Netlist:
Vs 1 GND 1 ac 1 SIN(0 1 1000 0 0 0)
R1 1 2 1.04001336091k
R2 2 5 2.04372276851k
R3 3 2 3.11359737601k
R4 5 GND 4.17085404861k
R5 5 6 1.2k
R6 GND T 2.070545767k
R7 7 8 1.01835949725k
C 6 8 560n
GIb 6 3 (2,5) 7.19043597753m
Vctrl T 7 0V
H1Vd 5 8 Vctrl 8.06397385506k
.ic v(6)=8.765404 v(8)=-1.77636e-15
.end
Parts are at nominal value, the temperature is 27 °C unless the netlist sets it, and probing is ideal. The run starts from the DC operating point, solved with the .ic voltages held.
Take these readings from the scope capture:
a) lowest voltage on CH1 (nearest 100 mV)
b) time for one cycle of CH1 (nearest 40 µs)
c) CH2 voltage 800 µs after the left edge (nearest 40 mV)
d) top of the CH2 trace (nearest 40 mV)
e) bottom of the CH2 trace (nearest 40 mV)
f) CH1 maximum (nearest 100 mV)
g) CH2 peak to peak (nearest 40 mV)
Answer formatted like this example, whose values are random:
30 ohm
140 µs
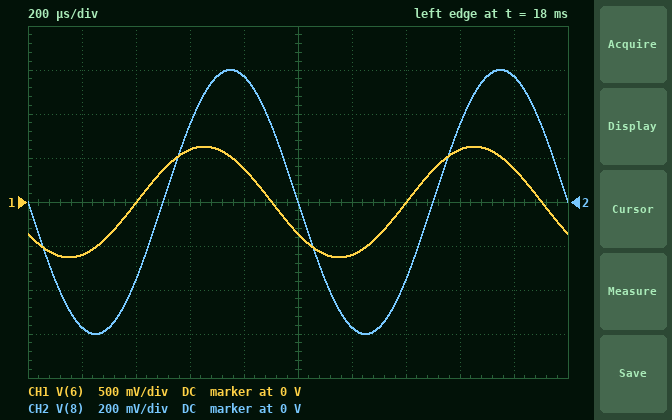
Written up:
-600 mV
1.00 ms
560 mV
600 mV
-600 mV
600 mV
1.20 V
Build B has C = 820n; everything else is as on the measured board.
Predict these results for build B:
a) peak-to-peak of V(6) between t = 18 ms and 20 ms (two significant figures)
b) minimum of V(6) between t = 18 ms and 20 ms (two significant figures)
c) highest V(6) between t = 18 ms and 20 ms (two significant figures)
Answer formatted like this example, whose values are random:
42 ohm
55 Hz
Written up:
1.2 V
-610 mV
610 mV
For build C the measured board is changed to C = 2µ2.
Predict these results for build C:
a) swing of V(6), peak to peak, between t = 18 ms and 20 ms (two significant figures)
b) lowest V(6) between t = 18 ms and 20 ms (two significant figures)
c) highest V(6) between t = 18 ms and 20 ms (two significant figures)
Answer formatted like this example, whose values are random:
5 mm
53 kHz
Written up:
1.2 V
-600 mV
610 mV
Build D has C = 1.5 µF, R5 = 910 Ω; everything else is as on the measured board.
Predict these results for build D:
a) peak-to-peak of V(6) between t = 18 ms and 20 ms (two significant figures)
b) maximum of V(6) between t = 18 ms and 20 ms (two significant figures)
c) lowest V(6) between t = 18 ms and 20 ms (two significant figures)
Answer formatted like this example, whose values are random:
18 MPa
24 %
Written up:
1.2 V
610 mV
-610 mV
